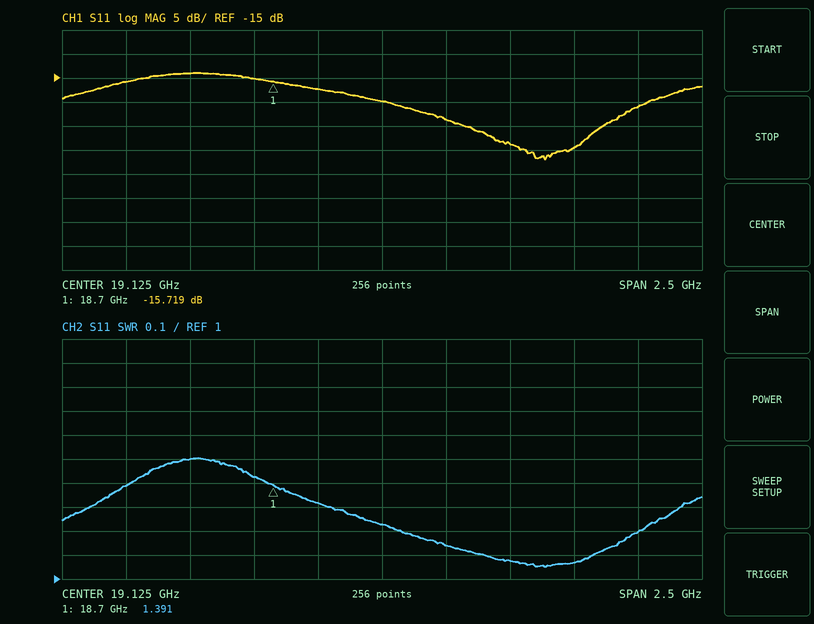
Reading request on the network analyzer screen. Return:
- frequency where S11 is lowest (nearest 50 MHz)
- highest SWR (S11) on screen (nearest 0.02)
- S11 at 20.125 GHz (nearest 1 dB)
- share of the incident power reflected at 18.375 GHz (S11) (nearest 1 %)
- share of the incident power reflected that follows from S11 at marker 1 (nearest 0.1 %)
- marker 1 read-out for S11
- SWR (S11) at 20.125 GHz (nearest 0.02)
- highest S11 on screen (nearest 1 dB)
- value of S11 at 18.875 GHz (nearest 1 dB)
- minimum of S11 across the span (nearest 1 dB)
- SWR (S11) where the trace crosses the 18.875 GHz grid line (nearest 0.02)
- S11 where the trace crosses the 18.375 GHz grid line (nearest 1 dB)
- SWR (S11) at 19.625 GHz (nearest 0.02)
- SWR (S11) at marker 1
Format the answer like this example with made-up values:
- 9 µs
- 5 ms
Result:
- 19.75 GHz
- 1.50
- -21 dB
- 4 %
- 2.7 %
- -15.719 dB
- 1.20
- -14 dB
- -17 dB
- -32 dB
- 1.32
- -14 dB
- 1.08
- 1.391
